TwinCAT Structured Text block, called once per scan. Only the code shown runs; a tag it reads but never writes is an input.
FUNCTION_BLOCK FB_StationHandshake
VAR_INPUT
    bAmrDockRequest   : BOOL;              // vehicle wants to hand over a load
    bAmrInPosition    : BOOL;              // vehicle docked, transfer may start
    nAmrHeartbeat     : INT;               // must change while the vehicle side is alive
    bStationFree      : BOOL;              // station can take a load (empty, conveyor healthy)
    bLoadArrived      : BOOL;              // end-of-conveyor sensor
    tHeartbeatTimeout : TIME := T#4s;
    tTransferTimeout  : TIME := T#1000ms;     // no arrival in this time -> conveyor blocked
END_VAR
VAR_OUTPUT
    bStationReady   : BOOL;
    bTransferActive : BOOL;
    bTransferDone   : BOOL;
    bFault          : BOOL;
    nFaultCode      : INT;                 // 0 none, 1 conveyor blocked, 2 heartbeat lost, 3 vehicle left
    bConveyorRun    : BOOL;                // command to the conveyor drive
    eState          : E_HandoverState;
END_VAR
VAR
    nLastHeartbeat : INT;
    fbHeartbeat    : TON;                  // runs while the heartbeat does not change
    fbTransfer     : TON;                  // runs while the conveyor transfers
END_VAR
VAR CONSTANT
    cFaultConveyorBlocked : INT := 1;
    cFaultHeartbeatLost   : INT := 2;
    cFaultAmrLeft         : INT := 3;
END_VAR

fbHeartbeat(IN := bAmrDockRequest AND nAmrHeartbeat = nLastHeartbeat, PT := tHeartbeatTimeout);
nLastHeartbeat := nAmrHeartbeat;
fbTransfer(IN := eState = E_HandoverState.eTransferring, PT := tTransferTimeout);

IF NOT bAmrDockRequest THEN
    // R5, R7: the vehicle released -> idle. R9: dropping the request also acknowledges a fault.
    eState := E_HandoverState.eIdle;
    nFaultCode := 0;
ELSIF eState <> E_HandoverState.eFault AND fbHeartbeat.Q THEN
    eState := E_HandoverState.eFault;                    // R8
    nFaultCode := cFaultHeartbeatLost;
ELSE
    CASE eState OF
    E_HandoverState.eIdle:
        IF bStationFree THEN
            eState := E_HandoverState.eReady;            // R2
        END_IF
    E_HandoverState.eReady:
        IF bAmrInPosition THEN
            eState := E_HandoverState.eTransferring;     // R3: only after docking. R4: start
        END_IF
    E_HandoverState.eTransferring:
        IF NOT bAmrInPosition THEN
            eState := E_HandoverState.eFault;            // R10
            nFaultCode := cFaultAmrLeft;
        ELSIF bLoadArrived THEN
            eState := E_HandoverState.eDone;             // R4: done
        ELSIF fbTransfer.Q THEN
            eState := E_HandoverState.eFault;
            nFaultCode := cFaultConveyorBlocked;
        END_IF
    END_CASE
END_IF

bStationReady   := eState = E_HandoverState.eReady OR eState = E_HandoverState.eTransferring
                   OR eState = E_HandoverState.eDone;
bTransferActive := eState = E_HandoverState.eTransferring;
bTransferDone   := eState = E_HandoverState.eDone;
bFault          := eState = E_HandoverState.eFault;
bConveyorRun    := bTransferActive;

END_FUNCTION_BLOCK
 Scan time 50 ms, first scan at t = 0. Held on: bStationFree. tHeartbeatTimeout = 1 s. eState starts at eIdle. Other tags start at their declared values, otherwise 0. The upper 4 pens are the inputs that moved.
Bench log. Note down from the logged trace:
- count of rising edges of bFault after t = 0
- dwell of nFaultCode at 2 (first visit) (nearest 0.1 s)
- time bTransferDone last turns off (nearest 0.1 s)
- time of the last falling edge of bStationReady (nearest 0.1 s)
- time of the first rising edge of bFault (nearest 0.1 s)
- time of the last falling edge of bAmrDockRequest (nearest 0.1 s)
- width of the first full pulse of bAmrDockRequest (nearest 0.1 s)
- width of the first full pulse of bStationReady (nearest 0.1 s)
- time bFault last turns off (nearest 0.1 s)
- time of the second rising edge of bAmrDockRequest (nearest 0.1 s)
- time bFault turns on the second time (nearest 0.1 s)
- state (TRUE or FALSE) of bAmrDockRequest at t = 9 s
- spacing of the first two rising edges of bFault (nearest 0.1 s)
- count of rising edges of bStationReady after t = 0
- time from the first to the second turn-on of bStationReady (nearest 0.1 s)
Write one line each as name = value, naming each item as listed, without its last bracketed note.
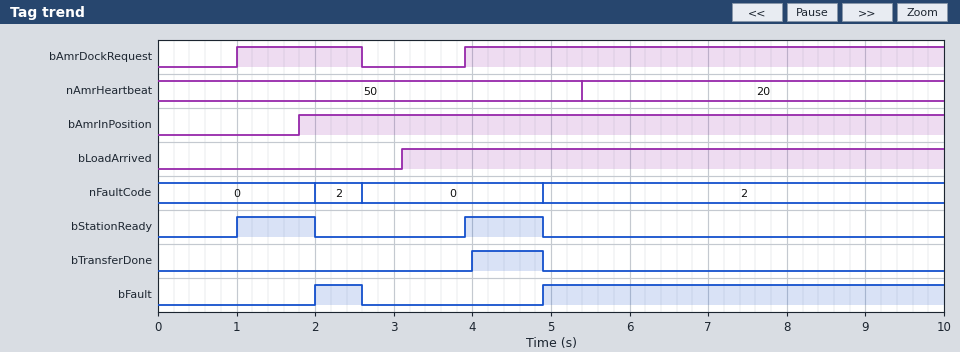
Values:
count of rising edges of bFault after t = 0 = 2
dwell of nFaultCode at 2 (first visit) = 0.6 s
time bTransferDone last turns off = 4.9 s
time of the last falling edge of bStationReady = 4.9 s
time of the first rising edge of bFault = 2.0 s
time of the last falling edge of bAmrDockRequest = 2.6 s
width of the first full pulse of bAmrDockRequest = 1.6 s
width of the first full pulse of bStationReady = 1.0 s
time bFault last turns off = 2.6 s
time of the second rising edge of bAmrDockRequest = 3.9 s
time bFault turns on the second time = 4.9 s
state (TRUE or FALSE) of bAmrDockRequest at t = 9 s = TRUE
spacing of the first two rising edges of bFault = 2.9 s
count of rising edges of bStationReady after t = 0 = 2
time from the first to the second turn-on of bStationReady = 2.9 s
